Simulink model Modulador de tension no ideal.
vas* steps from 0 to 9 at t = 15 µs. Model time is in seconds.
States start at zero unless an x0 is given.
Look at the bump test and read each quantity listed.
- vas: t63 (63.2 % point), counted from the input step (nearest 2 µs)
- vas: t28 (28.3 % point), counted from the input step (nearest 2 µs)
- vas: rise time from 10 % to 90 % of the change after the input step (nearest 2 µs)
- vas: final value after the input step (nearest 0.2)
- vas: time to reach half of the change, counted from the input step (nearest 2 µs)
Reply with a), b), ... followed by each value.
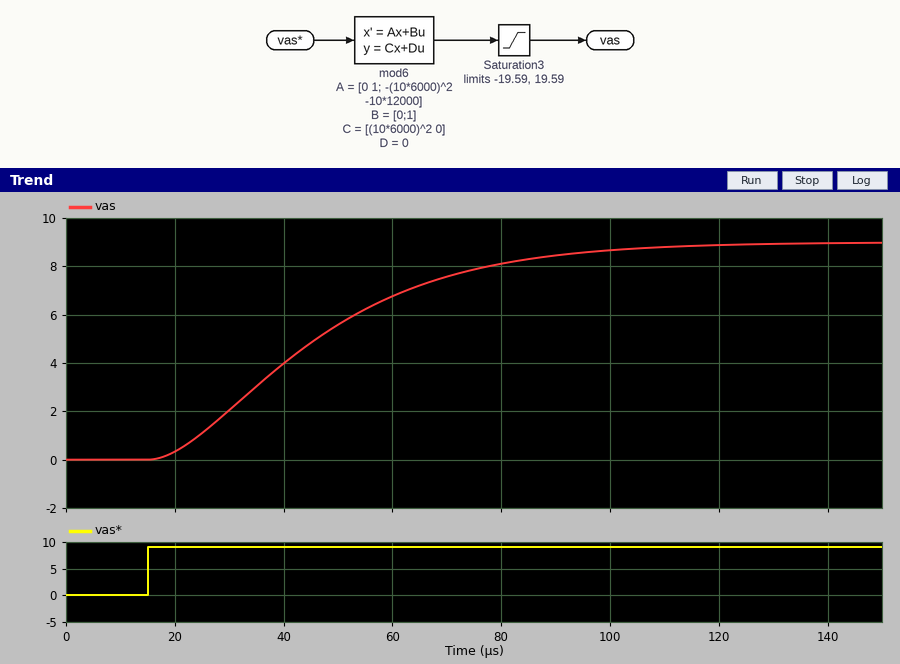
a) 36 µs
b) 18 µs
c) 56 µs
d) 9.0
e) 28 µs
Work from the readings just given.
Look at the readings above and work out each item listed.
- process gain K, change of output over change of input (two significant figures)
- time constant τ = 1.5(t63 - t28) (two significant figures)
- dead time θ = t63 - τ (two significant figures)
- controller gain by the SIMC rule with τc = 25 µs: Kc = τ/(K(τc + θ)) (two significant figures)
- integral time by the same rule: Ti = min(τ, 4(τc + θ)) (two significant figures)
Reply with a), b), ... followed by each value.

a) 1.0
b) 27 µs
c) 9.0 µs
d) 0.79
e) 27 µs
